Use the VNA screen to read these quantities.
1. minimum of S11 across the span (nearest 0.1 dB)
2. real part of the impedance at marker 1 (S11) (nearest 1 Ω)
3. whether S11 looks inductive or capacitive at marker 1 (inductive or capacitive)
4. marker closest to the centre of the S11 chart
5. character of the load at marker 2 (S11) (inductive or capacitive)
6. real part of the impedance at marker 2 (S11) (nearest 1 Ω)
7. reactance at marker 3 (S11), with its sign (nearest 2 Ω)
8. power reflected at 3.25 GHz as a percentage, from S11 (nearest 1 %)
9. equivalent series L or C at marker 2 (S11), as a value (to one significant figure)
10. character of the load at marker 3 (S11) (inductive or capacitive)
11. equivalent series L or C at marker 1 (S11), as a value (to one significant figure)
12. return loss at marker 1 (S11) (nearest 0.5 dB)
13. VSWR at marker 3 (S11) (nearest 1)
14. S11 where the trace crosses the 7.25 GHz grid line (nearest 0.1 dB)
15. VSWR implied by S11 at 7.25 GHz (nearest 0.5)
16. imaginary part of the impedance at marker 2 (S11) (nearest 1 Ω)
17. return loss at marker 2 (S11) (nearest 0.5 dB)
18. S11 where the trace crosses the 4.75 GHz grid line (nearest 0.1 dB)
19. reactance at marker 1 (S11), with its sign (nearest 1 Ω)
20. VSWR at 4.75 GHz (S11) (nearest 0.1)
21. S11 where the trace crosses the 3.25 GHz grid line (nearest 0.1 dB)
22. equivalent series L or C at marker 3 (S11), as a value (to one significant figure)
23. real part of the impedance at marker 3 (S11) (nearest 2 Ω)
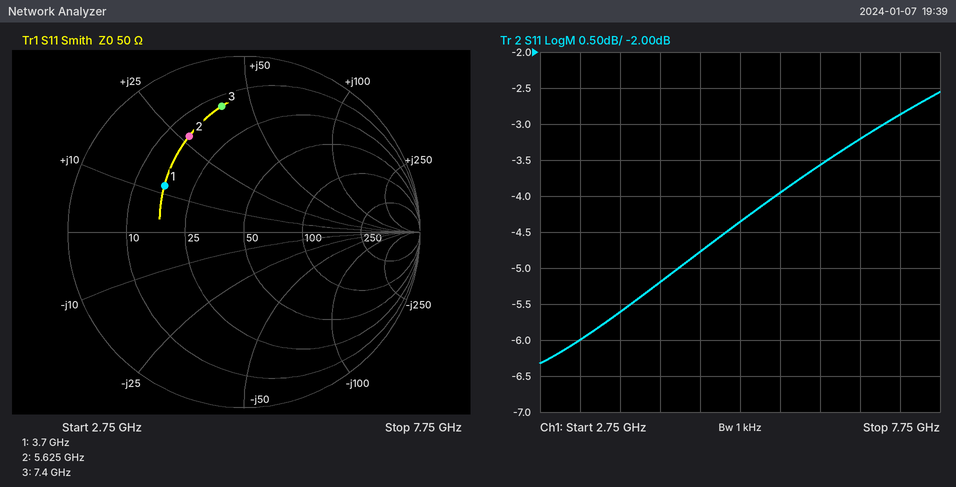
-6.3 dB
17 Ω
inductive
marker 1
inductive
15 Ω
+40 Ω
25 %
800 pH
inductive
500 pH
5.5 dB
6
-2.9 dB
6.0
+27 Ω
4.0 dB
-4.8 dB
+12 Ω
3.7
-6.0 dB
900 pH
14 Ω
